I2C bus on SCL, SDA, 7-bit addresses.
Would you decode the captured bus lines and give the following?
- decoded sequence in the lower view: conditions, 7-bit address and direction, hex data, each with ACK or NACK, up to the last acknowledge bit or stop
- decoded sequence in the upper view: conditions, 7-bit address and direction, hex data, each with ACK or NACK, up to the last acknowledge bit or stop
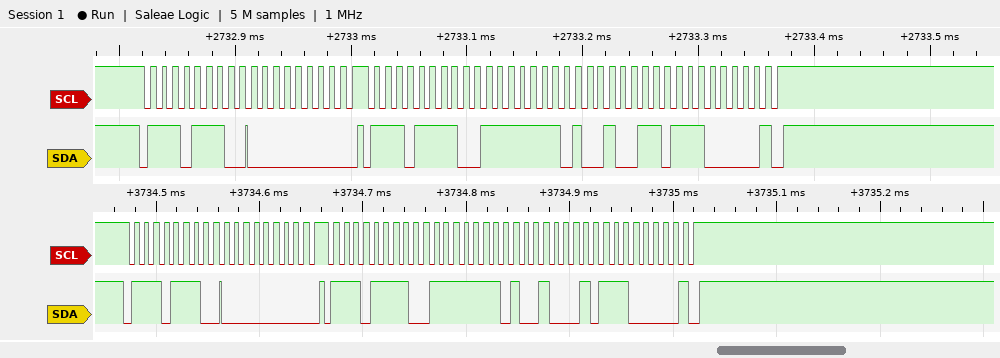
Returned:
start, address 77 write ACK, 00 ACK, stop, start, address 77 read ACK, 7F ACK, 91 ACK, E0 NACK, stop
start, address 77 write ACK, 00 ACK, stop, start, address 77 read ACK, 7F ACK, 93 ACK, E0 NACK, stop
